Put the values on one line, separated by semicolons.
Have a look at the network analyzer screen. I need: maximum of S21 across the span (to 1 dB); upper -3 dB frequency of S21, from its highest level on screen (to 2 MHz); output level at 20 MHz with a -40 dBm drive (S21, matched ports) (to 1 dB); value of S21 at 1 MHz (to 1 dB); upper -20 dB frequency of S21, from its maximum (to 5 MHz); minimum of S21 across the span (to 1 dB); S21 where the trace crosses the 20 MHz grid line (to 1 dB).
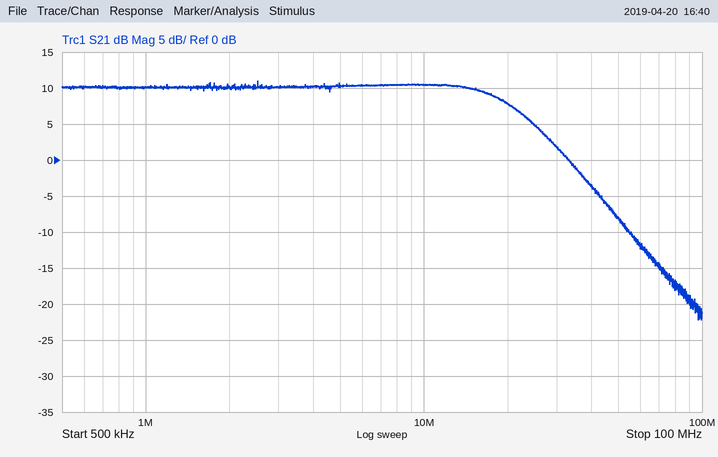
11 dB; 20 MHz; -32 dBm; 10 dB; 50 MHz; -22 dB; 8 dB
